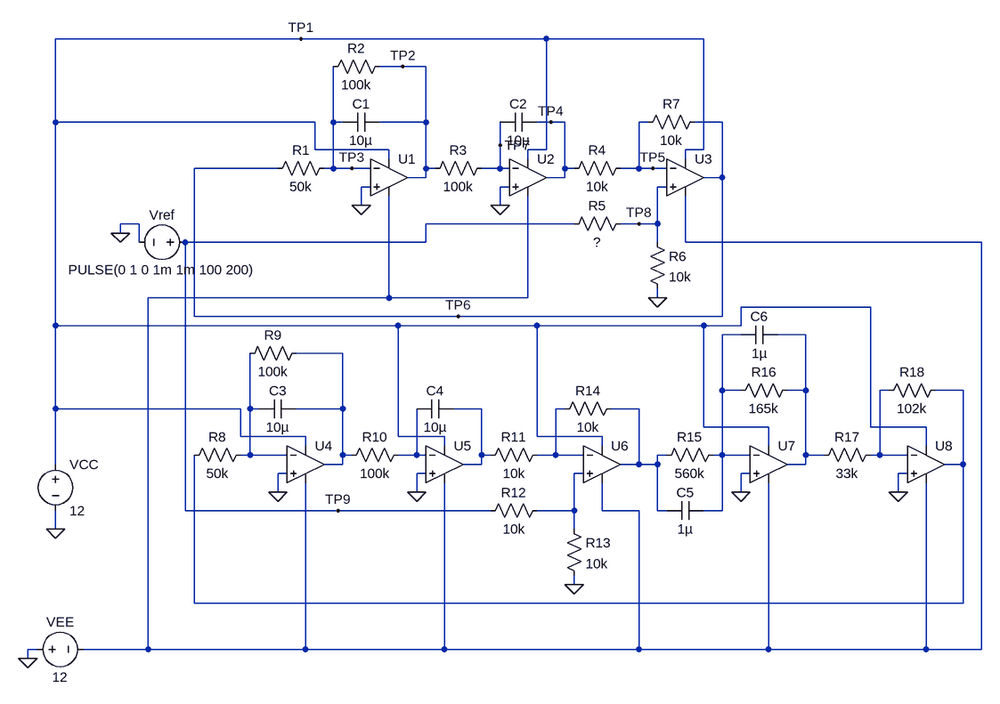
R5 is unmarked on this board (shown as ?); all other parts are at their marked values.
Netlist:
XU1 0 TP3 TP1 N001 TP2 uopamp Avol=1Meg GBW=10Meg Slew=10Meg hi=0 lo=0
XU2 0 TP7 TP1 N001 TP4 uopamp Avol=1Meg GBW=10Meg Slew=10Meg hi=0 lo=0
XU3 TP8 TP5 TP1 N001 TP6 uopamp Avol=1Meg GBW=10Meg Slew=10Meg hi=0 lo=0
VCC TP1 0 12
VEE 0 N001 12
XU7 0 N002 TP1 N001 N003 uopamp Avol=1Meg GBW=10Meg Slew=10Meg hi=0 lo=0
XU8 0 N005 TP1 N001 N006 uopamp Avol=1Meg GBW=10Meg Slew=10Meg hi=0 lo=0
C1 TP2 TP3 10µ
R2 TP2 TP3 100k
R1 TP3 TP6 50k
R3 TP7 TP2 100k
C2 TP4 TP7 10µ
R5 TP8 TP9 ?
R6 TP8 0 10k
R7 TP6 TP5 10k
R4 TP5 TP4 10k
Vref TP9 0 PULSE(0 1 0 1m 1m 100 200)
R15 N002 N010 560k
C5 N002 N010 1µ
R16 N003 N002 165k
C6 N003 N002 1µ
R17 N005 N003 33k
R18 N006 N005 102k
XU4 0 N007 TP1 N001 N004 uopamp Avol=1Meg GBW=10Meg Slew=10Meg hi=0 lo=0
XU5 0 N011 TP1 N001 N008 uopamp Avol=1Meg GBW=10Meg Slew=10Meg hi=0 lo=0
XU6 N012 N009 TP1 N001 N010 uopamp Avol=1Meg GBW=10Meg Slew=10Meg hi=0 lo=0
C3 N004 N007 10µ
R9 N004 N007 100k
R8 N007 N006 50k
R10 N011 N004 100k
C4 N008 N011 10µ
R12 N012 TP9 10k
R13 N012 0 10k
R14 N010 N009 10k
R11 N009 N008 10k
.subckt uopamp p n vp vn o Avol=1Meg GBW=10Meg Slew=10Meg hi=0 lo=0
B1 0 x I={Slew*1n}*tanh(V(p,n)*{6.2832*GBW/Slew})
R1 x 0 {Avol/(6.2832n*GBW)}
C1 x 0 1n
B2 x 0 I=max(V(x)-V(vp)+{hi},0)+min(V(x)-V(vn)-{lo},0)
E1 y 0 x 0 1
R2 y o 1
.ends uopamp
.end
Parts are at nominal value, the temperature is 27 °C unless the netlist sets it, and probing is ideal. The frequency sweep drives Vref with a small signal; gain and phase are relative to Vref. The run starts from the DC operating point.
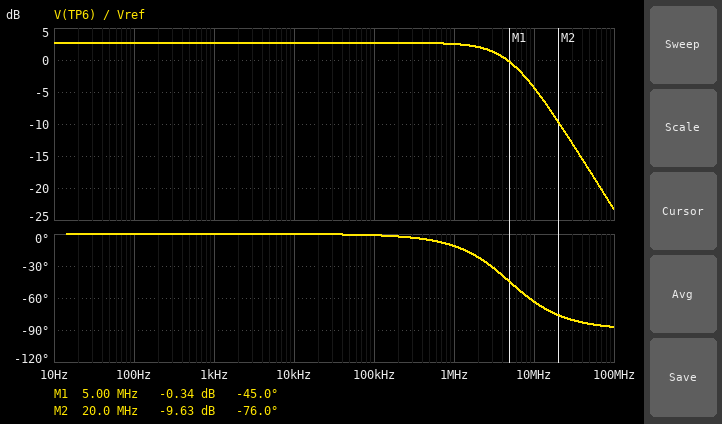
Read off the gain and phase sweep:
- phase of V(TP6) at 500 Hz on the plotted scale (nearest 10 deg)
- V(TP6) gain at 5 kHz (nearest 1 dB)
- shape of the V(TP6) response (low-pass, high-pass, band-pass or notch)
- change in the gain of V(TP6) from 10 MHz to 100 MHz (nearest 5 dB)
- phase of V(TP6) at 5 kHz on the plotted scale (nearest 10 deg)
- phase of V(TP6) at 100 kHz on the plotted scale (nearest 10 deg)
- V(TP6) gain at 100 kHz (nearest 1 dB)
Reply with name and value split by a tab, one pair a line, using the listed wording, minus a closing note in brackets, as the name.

phase of V(TP6) at 500 Hz on the plotted scale	0 deg
V(TP6) gain at 5 kHz	3 dB
shape of the V(TP6) response	low-pass
change in the gain of V(TP6) from 10 MHz to 100 MHz	-20 dB
phase of V(TP6) at 5 kHz on the plotted scale	0 deg
phase of V(TP6) at 100 kHz on the plotted scale	0 deg
V(TP6) gain at 100 kHz	3 dB
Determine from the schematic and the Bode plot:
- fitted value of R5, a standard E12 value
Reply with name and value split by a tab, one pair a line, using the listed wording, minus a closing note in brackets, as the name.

fitted value of R5, a standard E12 value	4.7 kΩ
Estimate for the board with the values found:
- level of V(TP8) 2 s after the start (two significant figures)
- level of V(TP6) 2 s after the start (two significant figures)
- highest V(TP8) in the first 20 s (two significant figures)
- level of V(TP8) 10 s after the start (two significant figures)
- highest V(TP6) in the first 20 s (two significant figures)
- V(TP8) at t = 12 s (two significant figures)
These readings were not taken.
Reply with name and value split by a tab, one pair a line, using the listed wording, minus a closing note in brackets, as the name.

level of V(TP8) 2 s after the start	680 mV
level of V(TP6) 2 s after the start	-350 mV
highest V(TP8) in the first 20 s	680 mV
level of V(TP8) 10 s after the start	680 mV
highest V(TP6) in the first 20 s	1.4 V
V(TP8) at t = 12 s	680 mV
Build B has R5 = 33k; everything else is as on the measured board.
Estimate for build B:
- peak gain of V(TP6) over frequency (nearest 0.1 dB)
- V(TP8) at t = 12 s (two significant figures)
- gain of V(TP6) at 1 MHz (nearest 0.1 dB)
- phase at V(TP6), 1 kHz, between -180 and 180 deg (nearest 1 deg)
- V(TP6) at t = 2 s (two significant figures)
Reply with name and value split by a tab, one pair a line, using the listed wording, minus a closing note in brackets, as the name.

peak gain of V(TP6) over frequency	-1.6 dB
V(TP8) at t = 12 s	230 mV
gain of V(TP6) at 1 MHz	-6.8 dB
phase at V(TP6), 1 kHz, between -180 and 180 deg	0 deg
V(TP6) at t = 2 s	-120 mV
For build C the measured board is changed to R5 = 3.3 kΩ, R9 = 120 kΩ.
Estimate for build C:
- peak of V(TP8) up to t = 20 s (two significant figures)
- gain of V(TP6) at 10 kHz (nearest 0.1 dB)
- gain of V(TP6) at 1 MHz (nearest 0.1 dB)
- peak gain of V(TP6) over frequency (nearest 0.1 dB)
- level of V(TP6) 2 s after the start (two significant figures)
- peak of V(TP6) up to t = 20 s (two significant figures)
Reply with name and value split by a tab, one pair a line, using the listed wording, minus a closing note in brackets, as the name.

peak of V(TP8) up to t = 20 s	750 mV
gain of V(TP6) at 10 kHz	3.5 dB
gain of V(TP6) at 1 MHz	3.4 dB
peak gain of V(TP6) over frequency	8.6 dB
level of V(TP6) 2 s after the start	-390 mV
peak of V(TP6) up to t = 20 s	1.5 V
